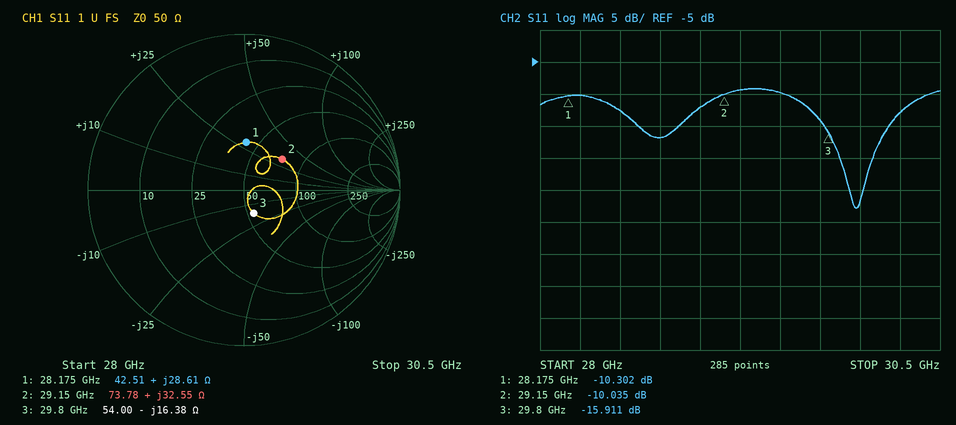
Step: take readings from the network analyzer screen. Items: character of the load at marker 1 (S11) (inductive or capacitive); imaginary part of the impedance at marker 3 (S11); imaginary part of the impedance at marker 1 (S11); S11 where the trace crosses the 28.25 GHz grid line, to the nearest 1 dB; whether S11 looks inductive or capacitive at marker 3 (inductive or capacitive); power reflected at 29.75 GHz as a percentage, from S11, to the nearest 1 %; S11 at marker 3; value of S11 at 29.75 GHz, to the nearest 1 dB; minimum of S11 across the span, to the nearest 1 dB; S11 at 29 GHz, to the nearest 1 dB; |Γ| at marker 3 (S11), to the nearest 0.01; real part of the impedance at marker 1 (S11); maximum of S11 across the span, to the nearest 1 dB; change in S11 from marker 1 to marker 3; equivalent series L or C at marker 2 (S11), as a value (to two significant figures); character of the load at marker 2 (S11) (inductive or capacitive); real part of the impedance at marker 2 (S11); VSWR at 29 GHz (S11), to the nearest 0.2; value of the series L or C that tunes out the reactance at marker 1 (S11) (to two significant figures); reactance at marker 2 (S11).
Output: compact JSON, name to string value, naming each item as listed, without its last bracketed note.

{"character of the load at marker 1 (S11)": "inductive", "imaginary part of the impedance at marker 3": "-16.38 Ω", "imaginary part of the impedance at marker 1": "+28.61 Ω", "S11 where the trace crosses the 28.25 GHz grid line, to the nearest 1 dB": "-10 dB", "whether S11 looks inductive or capacitive at marker 3": "capacitive", "power reflected at 29.75 GHz as a percentage, from S11, to the nearest 1 %": "4 %", "S11 at marker 3": "-15.911 dB", "value of S11 at 29.75 GHz, to the nearest 1 dB": "-14 dB", "minimum of S11 across the span, to the nearest 1 dB": "-28 dB", "S11 at 29 GHz, to the nearest 1 dB": "-12 dB", "|Γ| at marker 3 (S11), to the nearest 0.01": "0.16", "real part of the impedance at marker 1": "42.51 Ω", "maximum of S11 across the span, to the nearest 1 dB": "-9 dB", "change in S11 from marker 1 to marker 3": "-5.609 dB", "equivalent series L or C at marker 2 (S11), as a value": "180 pH", "character of the load at marker 2 (S11)": "inductive", "real part of the impedance at marker 2": "73.78 Ω", "VSWR at 29 GHz (S11), to the nearest 0.2": "1.6", "value of the series L or C that tunes out the reactance at marker 1 (S11)": "200 fF", "reactance at marker 2": "+32.55 Ω"}
